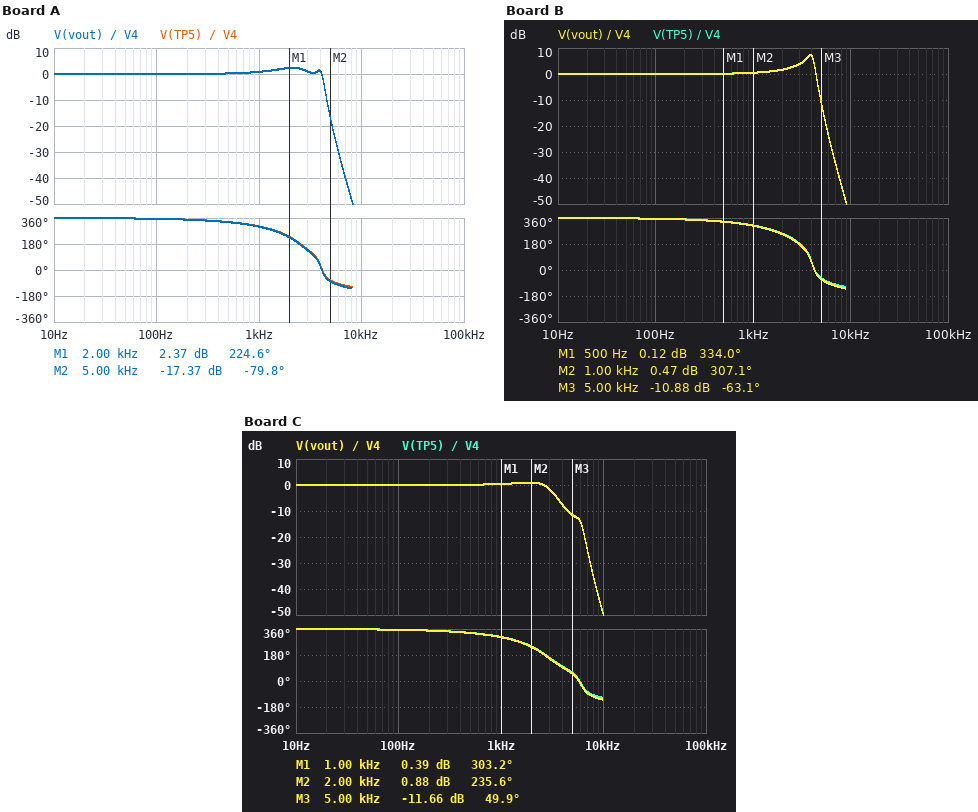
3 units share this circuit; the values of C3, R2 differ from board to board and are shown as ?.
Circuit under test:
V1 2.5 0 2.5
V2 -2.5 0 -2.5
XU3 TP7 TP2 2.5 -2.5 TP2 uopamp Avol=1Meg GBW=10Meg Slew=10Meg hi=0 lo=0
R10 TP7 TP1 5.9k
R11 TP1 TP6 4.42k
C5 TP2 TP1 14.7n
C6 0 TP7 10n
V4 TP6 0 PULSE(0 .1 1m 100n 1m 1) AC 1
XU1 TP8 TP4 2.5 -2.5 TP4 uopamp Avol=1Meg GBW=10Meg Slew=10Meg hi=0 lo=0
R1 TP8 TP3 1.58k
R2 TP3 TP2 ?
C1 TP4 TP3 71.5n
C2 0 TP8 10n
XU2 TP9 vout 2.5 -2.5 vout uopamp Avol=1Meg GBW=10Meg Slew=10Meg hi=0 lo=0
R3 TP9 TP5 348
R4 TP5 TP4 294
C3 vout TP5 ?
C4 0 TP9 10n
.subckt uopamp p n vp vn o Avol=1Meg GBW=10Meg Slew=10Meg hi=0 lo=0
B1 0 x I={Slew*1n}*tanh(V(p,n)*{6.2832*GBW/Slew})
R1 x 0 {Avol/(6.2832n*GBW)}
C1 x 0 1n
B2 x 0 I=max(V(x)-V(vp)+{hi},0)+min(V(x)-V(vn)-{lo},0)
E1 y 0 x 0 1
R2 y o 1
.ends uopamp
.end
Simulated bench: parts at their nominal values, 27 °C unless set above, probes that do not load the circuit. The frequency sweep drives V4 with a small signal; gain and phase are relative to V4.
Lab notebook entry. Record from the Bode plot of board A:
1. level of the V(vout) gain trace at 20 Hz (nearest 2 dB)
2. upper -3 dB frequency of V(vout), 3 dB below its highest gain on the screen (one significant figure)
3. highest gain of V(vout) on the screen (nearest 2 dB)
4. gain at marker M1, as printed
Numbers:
0 dB
4 kHz
2 dB
2.37 dB
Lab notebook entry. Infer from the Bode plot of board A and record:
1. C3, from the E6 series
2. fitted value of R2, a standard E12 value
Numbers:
1.5 µF
3.3 kΩ
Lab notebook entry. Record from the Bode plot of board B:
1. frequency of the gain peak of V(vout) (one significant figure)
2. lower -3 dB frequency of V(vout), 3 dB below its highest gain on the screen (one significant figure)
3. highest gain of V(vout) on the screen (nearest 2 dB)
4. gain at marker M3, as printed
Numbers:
4 kHz
3 kHz
8 dB
-10.88 dB
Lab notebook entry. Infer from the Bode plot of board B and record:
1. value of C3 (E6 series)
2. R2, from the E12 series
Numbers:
1.5 µF
1.8 kΩ
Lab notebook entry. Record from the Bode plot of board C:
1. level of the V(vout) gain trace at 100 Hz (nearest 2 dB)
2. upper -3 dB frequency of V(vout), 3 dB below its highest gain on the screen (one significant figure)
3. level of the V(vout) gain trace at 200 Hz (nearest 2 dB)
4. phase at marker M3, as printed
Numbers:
0 dB
3 kHz
0 dB
49.9 deg
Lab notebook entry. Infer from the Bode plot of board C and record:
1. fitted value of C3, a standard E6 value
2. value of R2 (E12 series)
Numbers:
680 nF
2.7 kΩ
